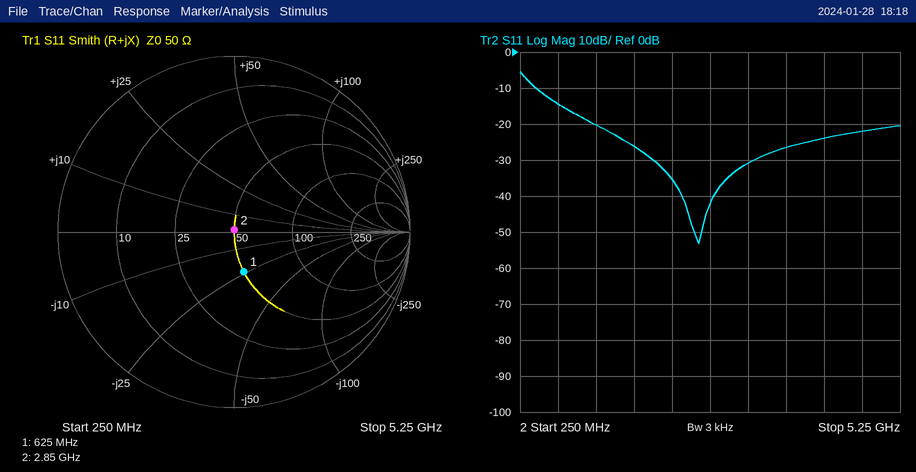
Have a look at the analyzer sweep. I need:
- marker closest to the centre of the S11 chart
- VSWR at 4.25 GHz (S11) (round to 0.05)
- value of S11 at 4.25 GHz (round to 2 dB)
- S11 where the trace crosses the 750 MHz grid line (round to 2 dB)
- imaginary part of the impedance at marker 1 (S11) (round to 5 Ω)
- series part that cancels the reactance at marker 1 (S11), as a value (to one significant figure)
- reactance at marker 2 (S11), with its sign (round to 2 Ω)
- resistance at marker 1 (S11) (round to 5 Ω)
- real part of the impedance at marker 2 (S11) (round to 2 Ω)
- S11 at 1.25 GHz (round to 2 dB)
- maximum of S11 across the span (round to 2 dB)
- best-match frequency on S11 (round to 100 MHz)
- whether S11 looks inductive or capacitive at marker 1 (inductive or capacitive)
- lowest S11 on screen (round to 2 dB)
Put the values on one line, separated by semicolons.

marker 2; 1.15; -24 dB; -14 dB; -25 Ω; 6 nH; +2 Ω; 50 Ω; 50 Ω; -20 dB; -6 dB; 2.6 GHz; capacitive; -54 dB
